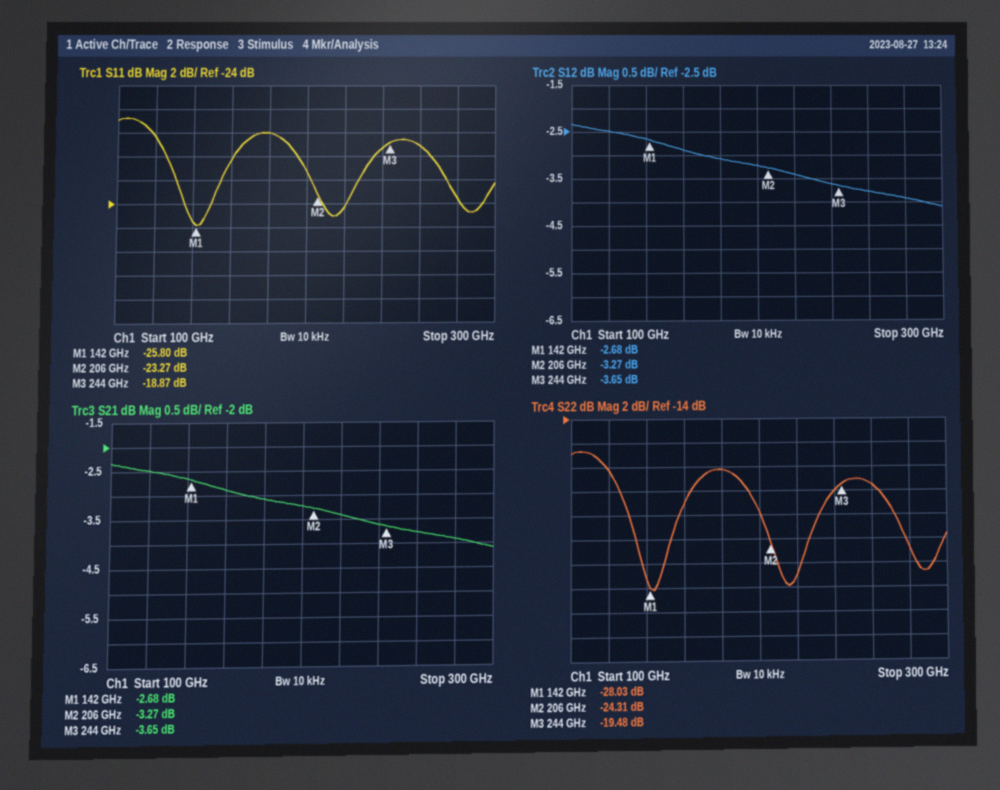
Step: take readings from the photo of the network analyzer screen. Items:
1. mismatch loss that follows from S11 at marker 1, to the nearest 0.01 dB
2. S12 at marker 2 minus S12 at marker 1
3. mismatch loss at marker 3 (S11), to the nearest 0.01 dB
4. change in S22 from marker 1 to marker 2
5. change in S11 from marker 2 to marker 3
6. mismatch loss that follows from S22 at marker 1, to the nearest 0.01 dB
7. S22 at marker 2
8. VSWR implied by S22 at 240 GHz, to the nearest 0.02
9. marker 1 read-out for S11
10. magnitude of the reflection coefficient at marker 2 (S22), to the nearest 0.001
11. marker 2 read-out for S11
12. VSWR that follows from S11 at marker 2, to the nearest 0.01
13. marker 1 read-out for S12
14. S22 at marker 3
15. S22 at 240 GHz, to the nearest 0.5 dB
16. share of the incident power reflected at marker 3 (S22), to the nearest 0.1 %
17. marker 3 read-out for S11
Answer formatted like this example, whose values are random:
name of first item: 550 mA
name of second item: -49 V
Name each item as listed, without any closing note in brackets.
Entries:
mismatch loss that follows from S11 at marker 1, to the nearest 0.01 dB: 0.01 dB
S12 at marker 2 minus S12 at marker 1: -0.59 dB
mismatch loss at marker 3 (S11), to the nearest 0.01 dB: 0.06 dB
change in S22 from marker 1 to marker 2: 3.72 dB
change in S11 from marker 2 to marker 3: 4.40 dB
mismatch loss that follows from S22 at marker 1, to the nearest 0.01 dB: 0.01 dB
S22 at marker 2: -24.31 dB
VSWR implied by S22 at 240 GHz, to the nearest 0.02: 1.22
marker 1 read-out for S11: -25.80 dB
magnitude of the reflection coefficient at marker 2 (S22), to the nearest 0.001: 0.061
marker 2 read-out for S11: -23.27 dB
VSWR that follows from S11 at marker 2, to the nearest 0.01: 1.15
marker 1 read-out for S12: -2.68 dB
S22 at marker 3: -19.48 dB
S22 at 240 GHz, to the nearest 0.5 dB: -20.0 dB
share of the incident power reflected at marker 3 (S22), to the nearest 0.1 %: 1.1 %
marker 3 read-out for S11: -18.87 dB
